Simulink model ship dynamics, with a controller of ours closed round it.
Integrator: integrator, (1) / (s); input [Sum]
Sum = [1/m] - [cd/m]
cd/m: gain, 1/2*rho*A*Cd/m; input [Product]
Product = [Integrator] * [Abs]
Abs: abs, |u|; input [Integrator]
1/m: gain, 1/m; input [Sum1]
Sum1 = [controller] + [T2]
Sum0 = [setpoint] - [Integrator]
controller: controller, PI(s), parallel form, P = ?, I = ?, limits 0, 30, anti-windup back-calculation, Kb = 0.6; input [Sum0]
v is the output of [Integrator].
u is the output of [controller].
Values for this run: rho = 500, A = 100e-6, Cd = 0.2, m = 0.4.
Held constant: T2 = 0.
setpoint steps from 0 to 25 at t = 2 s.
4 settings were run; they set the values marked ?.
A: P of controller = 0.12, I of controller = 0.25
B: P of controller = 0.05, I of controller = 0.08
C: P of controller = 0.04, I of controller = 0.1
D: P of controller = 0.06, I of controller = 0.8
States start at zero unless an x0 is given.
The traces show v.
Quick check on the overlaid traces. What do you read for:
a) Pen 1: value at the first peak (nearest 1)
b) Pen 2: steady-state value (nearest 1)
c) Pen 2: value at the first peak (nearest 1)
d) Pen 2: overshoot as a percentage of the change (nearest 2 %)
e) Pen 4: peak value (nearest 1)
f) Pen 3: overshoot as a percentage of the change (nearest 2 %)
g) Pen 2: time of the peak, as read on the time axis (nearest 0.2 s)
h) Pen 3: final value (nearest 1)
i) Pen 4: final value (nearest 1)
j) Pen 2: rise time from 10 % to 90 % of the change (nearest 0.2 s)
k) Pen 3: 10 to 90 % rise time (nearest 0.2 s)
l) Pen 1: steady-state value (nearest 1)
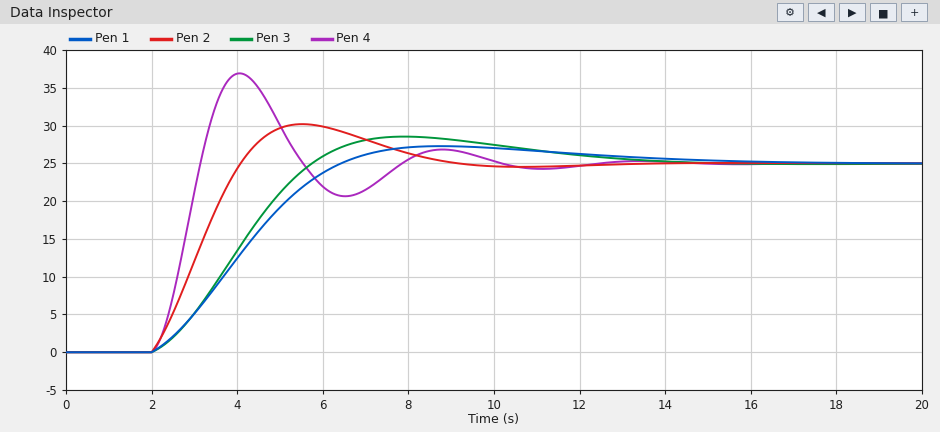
27
25
30
20 %
37
14 %
5.6 s
25
25
1.6 s
2.6 s
25
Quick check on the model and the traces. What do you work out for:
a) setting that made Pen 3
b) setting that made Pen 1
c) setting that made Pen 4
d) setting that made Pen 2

C
B
D
A
